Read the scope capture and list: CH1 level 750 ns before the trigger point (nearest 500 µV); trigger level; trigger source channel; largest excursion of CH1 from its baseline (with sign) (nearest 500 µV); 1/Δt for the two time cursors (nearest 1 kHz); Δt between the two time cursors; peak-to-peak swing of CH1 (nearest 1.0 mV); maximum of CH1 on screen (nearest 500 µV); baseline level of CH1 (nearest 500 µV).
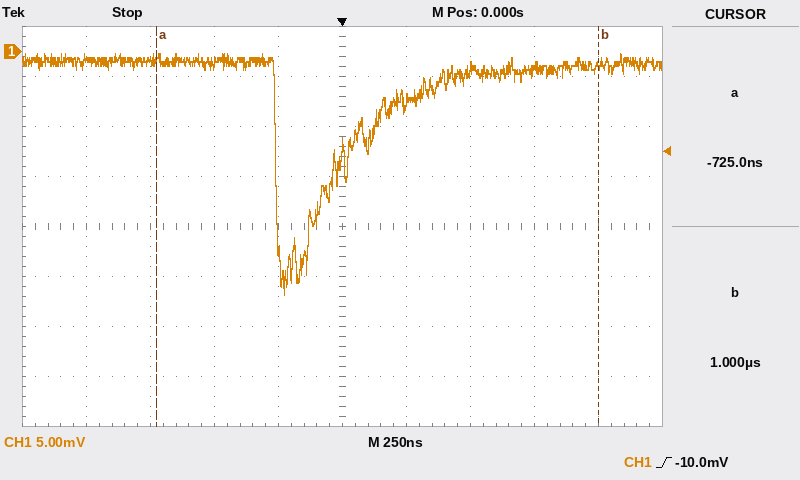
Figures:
-1.0 mV
-10.0 mV
CH1
-23.0 mV
580 kHz
1.725 µs
24.0 mV
0.0 mV
-1.0 mV
